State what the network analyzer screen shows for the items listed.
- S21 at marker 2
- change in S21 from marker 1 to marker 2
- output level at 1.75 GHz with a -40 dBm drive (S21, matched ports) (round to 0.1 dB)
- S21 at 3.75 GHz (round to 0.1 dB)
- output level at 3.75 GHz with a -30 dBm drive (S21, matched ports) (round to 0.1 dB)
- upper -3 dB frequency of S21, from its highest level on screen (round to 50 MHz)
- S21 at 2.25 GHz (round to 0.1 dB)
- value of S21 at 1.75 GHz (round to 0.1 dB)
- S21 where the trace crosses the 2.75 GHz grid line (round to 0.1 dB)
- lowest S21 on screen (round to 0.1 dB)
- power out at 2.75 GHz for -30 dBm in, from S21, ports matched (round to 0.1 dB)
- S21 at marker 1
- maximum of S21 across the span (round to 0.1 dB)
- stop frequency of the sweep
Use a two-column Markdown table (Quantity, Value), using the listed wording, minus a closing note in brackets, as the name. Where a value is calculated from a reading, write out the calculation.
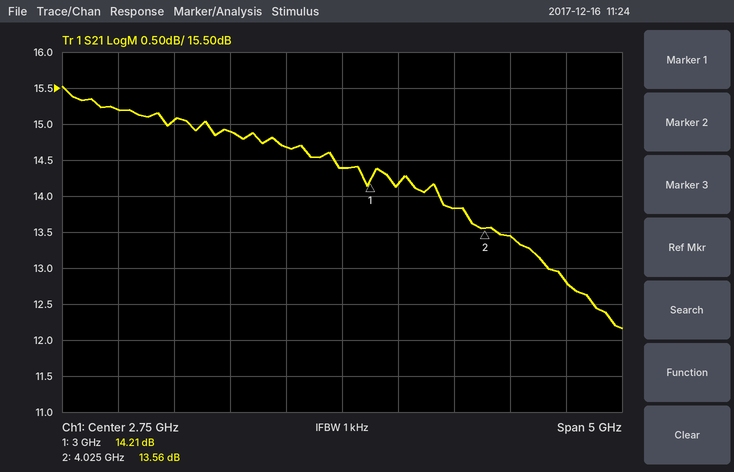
| Quantity | Value |
|---|---|
| S21 at marker 2 | 13.56 dB |
| change in S21 from marker 1 to marker 2 | 13.56 − (14.21) = -0.65 dB |
| output level at 1.75 GHz with a -40 dBm drive (S21, matched ports) | -40 dBm + (14.9 dB) = -25.1 dBm |
| S21 at 3.75 GHz | 13.8 dB |
| output level at 3.75 GHz with a -30 dBm drive (S21, matched ports) | -30 dBm + (13.8 dB) = -16.2 dBm |
| upper -3 dB frequency of S21, from its highest level on screen | 5.00 GHz |
| S21 at 2.25 GHz | 14.7 dB |
| value of S21 at 1.75 GHz | 14.9 dB |
| S21 where the trace crosses the 2.75 GHz grid line | 14.4 dB |
| lowest S21 on screen | 12.2 dB |
| power out at 2.75 GHz for -30 dBm in, from S21, ports matched | -30 dBm + (14.4 dB) = -15.6 dBm |
| S21 at marker 1 | 14.21 dB |
| maximum of S21 across the span | 15.5 dB |
| stop frequency of the sweep | 5.25 GHz |
